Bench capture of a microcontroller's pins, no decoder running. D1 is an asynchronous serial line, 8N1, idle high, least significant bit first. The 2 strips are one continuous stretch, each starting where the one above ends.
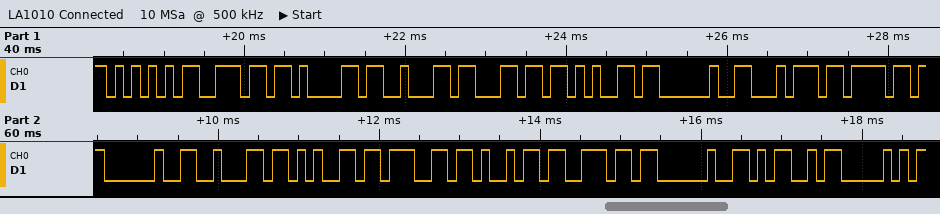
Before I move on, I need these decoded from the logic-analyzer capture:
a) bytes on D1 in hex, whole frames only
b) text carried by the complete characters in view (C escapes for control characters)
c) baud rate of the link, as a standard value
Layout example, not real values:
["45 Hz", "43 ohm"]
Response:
["55 6E 61 62 6C 65 20 74 6F 20 62 65 67 69 6E 20 4D 50", "\"Unable to begin MP\"", "9600 baud"]
